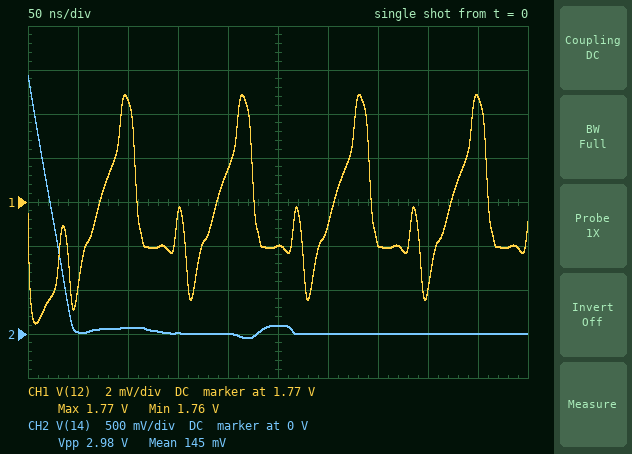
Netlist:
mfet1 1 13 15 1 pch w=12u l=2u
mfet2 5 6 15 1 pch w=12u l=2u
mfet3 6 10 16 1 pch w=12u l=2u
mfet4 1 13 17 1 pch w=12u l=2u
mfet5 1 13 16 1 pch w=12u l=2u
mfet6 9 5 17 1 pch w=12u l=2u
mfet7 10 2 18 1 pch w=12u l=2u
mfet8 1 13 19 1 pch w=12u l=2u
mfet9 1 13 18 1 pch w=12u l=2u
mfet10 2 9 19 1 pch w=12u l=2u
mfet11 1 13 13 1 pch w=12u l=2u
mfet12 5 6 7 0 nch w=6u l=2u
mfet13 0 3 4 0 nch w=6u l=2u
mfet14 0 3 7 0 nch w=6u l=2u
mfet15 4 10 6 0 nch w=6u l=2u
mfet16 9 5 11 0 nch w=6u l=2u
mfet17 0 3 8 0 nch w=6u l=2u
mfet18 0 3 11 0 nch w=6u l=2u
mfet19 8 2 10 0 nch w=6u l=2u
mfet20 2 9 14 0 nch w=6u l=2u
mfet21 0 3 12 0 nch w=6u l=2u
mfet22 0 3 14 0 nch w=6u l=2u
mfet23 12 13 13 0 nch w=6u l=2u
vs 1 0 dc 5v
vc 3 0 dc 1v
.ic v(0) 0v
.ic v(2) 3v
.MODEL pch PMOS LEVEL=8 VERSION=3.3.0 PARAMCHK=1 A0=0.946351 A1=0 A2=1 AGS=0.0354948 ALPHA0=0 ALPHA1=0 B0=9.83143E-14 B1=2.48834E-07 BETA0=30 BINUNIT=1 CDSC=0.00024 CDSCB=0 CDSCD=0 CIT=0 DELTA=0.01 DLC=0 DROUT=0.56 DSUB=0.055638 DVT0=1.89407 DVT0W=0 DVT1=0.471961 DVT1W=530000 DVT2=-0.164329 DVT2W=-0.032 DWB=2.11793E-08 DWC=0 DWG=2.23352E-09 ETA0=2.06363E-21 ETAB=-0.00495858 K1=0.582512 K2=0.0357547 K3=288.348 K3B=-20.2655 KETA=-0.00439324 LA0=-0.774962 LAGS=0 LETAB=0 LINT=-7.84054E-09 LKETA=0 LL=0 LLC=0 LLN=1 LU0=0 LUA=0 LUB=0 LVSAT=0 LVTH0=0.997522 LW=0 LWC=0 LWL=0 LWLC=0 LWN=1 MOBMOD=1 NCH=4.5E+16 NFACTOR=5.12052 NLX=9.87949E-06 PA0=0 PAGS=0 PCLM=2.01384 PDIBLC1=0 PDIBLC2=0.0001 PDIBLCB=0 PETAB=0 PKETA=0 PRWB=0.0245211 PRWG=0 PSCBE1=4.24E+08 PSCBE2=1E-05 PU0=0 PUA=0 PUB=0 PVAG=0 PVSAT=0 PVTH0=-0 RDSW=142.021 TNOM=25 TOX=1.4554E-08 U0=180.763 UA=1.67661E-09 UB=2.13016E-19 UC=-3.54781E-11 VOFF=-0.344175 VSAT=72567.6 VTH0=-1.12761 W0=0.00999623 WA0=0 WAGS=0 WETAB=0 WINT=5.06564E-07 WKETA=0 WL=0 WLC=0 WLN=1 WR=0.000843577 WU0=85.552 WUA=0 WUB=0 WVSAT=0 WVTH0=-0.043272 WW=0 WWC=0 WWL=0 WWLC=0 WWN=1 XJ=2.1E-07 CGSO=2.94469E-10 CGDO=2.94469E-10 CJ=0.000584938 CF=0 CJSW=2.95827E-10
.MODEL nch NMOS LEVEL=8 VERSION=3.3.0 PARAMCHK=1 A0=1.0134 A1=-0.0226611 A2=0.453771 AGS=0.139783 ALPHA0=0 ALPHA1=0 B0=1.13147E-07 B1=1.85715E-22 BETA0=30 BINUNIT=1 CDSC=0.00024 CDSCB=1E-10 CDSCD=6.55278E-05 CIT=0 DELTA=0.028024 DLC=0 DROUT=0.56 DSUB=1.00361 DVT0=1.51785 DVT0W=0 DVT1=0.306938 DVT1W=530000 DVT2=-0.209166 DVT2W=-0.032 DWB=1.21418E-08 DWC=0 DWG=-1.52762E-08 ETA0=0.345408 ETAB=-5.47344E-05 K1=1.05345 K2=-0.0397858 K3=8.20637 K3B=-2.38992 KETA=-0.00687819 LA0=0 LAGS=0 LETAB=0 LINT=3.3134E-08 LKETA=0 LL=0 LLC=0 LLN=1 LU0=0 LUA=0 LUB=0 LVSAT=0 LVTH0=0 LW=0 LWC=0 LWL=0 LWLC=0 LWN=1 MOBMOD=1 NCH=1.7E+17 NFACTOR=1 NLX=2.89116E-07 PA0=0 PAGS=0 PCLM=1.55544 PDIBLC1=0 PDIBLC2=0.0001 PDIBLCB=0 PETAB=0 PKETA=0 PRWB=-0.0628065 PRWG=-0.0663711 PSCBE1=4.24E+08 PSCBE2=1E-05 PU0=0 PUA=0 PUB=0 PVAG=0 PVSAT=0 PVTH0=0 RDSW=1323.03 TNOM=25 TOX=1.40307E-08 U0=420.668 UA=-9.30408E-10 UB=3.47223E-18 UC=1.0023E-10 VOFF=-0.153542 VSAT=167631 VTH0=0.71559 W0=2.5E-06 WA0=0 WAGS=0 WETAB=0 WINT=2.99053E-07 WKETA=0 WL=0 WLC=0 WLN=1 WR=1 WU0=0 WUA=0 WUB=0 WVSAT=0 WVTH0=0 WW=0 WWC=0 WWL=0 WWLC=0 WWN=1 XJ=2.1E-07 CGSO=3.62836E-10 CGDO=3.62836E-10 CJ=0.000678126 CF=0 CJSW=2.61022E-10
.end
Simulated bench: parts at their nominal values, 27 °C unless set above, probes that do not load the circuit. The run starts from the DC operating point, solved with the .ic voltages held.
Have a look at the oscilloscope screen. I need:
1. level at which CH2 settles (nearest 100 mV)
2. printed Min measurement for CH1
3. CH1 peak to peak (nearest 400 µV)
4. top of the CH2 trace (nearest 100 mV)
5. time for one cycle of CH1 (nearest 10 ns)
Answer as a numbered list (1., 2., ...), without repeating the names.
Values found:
1. 0 V
2. 1.76 V
3. 10.4 mV
4. 2.9 V
5. 120 ns
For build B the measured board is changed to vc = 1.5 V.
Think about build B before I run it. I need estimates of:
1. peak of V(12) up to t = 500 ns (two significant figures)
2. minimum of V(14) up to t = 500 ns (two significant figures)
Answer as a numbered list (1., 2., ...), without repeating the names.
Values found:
1. 960 mV
2. -120 mV
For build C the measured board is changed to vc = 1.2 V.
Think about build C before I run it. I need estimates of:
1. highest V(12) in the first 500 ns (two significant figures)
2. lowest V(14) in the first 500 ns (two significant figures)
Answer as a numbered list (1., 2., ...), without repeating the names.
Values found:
1. 1.4 V
2. -80 mV
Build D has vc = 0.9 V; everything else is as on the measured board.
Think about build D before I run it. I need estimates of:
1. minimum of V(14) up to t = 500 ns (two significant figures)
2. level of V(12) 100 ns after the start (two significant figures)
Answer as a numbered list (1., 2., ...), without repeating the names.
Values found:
1. -2.1 mV
2. 1.9 V
